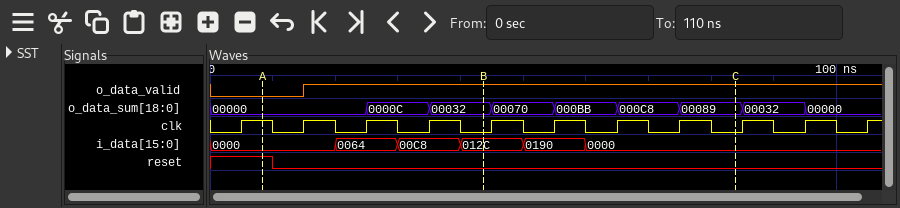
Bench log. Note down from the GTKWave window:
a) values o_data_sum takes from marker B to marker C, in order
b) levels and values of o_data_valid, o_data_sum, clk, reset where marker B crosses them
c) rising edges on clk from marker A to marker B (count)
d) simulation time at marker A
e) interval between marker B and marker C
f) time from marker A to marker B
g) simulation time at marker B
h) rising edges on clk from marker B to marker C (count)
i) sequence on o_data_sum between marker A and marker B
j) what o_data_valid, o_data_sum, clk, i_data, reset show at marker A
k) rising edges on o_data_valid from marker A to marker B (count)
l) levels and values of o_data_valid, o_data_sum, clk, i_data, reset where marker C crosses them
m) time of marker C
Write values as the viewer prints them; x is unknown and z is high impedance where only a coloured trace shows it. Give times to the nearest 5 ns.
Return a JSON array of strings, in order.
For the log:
["00032, 00070, 000BB, 000C8, 00089", "o_data_valid=1, o_data_sum=00032, clk=0, reset=0", "3", "10 ns", "40 ns", "35 ns", "45 ns", "4", "00000, 0000C, 00032", "o_data_valid=0, o_data_sum=00000, clk=1, i_data=0000, reset=1", "1", "o_data_valid=1, o_data_sum=00089, clk=0, i_data=0000, reset=0", "85 ns"]
